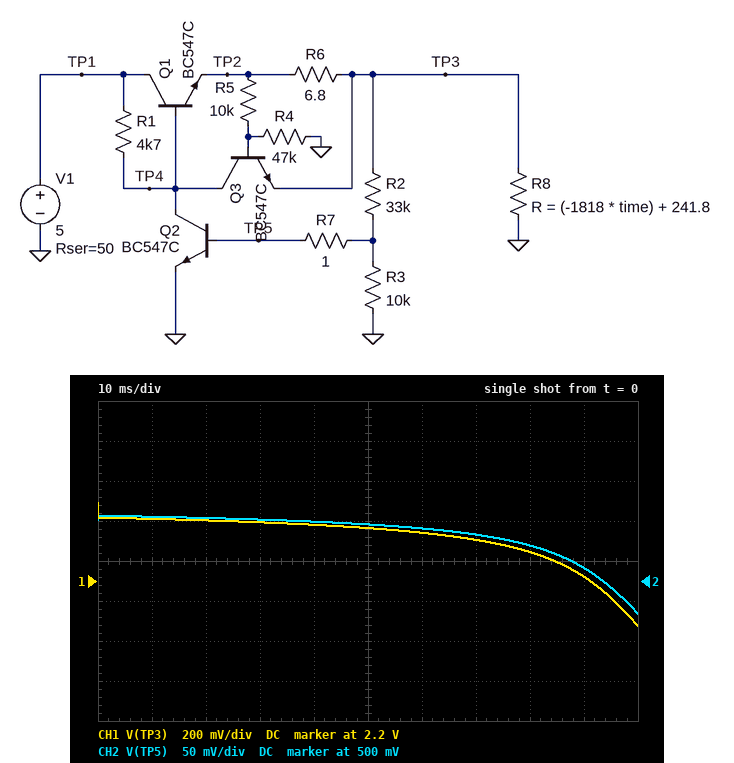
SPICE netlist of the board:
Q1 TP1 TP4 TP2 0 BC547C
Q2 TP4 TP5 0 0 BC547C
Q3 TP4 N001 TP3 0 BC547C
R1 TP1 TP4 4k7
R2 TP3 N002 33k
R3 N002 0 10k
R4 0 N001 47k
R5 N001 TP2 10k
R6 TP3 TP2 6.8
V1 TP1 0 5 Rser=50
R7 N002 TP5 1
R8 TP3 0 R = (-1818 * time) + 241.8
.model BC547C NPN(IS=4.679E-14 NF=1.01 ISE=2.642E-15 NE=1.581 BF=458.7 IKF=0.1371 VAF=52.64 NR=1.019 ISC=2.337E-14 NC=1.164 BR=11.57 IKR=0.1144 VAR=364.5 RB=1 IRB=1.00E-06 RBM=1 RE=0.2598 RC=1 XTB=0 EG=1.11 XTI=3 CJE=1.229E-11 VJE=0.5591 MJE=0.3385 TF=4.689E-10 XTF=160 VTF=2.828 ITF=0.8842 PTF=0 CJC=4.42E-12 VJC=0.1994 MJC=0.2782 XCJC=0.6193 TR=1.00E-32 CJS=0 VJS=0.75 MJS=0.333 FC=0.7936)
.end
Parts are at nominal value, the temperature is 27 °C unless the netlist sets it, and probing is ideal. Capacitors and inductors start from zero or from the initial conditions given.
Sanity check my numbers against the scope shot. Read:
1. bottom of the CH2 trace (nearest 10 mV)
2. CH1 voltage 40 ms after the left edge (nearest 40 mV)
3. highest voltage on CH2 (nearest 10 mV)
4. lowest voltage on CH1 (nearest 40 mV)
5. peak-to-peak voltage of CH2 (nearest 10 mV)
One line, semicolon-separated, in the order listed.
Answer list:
460 mV; 2.48 V; 580 mV; 1.96 V; 120 mV
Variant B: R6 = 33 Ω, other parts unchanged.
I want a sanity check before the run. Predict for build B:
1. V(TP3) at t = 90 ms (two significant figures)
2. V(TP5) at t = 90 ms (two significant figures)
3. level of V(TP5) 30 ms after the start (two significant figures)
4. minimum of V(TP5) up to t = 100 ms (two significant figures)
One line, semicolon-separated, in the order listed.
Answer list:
1.9 V; 450 mV; 570 mV; 380 mV
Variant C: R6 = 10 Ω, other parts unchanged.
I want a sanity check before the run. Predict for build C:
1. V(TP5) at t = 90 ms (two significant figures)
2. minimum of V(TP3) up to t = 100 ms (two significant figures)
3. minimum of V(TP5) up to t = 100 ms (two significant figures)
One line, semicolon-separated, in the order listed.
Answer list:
510 mV; 1.9 V; 450 mV
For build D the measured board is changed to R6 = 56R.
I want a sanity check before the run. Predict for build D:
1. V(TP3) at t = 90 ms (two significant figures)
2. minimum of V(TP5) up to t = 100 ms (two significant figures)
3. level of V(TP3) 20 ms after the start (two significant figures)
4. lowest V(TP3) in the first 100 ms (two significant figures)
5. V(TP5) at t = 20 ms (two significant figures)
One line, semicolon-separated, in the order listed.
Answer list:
1.4 V; 240 mV; 2.4 V; 1.0 V; 560 mV
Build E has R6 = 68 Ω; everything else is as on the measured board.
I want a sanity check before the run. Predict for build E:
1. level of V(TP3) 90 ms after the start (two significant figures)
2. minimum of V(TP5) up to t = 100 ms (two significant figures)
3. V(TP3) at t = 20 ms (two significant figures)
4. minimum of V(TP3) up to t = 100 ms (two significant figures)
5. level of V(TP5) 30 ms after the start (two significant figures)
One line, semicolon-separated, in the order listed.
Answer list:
1.1 V; 190 mV; 2.4 V; 820 mV; 550 mV
